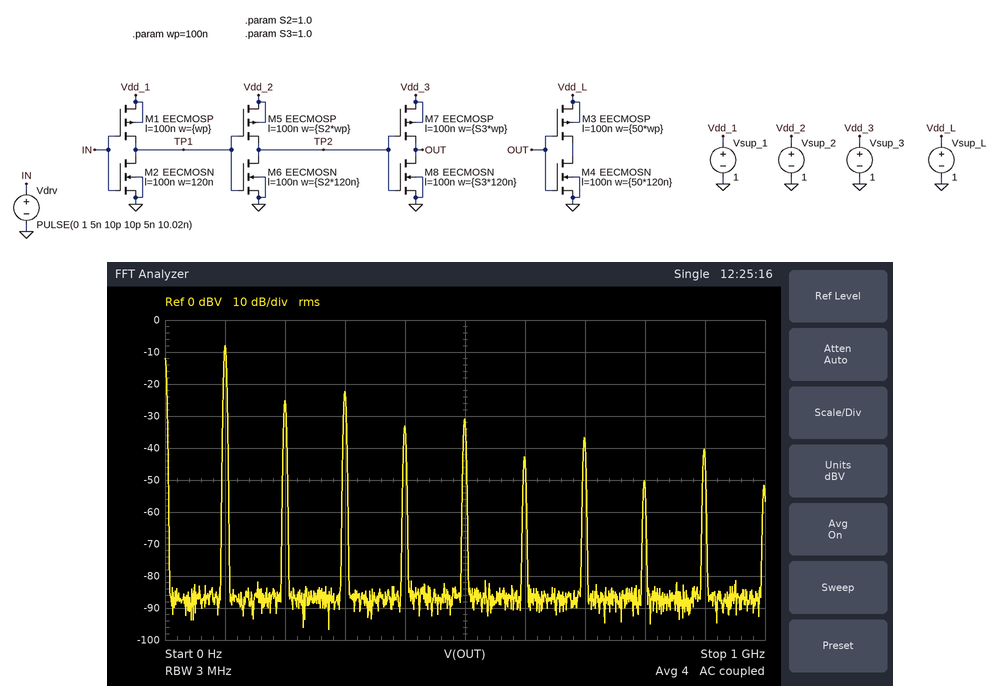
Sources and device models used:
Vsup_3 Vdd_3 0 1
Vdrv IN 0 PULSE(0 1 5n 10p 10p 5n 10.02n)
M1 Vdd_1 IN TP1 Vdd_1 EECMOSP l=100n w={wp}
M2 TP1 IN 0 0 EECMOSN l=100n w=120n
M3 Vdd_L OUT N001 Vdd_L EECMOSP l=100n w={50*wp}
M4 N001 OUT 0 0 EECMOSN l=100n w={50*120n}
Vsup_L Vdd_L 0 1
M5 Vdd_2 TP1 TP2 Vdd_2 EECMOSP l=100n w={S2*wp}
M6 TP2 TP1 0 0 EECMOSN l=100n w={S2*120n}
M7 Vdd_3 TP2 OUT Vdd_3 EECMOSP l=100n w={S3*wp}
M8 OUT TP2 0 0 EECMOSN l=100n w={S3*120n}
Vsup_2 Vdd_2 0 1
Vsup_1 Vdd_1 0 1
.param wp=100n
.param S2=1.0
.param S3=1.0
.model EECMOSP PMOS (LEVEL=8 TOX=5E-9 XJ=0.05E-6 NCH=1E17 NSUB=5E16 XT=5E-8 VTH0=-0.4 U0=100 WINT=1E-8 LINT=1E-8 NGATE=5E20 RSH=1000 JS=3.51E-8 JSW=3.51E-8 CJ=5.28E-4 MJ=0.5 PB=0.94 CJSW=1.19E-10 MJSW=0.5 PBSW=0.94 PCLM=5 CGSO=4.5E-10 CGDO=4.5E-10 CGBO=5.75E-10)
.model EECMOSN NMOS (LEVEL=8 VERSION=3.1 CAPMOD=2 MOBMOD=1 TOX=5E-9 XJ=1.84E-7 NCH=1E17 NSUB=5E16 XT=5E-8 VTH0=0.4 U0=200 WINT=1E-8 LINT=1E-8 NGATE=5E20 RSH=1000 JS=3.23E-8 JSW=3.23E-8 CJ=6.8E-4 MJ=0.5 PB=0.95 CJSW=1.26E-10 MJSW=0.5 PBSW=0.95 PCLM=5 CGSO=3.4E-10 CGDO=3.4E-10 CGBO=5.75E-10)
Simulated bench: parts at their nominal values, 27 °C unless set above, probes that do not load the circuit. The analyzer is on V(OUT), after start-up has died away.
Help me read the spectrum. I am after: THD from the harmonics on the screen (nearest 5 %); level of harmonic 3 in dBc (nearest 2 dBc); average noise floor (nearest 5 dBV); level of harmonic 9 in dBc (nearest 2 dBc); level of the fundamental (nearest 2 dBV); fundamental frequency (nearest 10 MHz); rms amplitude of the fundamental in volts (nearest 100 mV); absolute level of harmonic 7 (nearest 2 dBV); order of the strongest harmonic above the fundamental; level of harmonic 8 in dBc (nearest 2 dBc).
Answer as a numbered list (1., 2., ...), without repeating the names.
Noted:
1. 25 %
2. -14 dBc
3. -85 dBV
4. -32 dBc
5. -8 dBV
6. 100 MHz
7. 400 mV
8. -36 dBV
9. 3
10. -42 dBc
